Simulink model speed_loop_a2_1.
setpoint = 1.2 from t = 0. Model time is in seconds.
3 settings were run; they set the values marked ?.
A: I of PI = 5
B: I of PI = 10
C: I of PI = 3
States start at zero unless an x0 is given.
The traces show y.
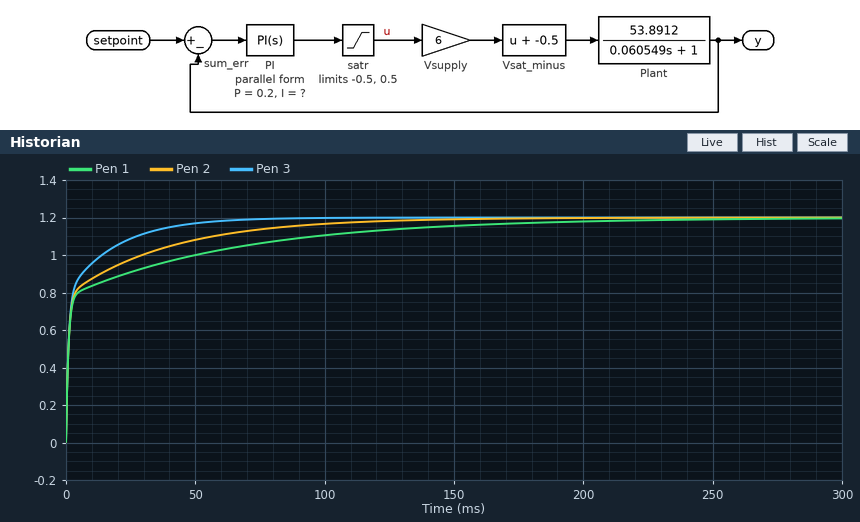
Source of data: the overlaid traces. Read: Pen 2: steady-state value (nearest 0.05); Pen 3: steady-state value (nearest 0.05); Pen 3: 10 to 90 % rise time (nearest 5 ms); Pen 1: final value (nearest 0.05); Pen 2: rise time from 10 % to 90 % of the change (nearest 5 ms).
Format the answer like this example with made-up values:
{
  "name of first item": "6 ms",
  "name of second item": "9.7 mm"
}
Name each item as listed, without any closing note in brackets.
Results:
{
  "Pen 2: steady-state value": "1.20",
  "Pen 3: steady-state value": "1.20",
  "Pen 3: 10 to 90 % rise time": "25 ms",
  "Pen 1: final value": "1.20",
  "Pen 2: rise time from 10 % to 90 % of the change": "50 ms"
}
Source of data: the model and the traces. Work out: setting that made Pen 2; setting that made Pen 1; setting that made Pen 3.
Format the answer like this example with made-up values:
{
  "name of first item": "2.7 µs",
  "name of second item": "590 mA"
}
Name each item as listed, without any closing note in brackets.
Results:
{
  "setting that made Pen 2": "A",
  "setting that made Pen 1": "C",
  "setting that made Pen 3": "B"
}
